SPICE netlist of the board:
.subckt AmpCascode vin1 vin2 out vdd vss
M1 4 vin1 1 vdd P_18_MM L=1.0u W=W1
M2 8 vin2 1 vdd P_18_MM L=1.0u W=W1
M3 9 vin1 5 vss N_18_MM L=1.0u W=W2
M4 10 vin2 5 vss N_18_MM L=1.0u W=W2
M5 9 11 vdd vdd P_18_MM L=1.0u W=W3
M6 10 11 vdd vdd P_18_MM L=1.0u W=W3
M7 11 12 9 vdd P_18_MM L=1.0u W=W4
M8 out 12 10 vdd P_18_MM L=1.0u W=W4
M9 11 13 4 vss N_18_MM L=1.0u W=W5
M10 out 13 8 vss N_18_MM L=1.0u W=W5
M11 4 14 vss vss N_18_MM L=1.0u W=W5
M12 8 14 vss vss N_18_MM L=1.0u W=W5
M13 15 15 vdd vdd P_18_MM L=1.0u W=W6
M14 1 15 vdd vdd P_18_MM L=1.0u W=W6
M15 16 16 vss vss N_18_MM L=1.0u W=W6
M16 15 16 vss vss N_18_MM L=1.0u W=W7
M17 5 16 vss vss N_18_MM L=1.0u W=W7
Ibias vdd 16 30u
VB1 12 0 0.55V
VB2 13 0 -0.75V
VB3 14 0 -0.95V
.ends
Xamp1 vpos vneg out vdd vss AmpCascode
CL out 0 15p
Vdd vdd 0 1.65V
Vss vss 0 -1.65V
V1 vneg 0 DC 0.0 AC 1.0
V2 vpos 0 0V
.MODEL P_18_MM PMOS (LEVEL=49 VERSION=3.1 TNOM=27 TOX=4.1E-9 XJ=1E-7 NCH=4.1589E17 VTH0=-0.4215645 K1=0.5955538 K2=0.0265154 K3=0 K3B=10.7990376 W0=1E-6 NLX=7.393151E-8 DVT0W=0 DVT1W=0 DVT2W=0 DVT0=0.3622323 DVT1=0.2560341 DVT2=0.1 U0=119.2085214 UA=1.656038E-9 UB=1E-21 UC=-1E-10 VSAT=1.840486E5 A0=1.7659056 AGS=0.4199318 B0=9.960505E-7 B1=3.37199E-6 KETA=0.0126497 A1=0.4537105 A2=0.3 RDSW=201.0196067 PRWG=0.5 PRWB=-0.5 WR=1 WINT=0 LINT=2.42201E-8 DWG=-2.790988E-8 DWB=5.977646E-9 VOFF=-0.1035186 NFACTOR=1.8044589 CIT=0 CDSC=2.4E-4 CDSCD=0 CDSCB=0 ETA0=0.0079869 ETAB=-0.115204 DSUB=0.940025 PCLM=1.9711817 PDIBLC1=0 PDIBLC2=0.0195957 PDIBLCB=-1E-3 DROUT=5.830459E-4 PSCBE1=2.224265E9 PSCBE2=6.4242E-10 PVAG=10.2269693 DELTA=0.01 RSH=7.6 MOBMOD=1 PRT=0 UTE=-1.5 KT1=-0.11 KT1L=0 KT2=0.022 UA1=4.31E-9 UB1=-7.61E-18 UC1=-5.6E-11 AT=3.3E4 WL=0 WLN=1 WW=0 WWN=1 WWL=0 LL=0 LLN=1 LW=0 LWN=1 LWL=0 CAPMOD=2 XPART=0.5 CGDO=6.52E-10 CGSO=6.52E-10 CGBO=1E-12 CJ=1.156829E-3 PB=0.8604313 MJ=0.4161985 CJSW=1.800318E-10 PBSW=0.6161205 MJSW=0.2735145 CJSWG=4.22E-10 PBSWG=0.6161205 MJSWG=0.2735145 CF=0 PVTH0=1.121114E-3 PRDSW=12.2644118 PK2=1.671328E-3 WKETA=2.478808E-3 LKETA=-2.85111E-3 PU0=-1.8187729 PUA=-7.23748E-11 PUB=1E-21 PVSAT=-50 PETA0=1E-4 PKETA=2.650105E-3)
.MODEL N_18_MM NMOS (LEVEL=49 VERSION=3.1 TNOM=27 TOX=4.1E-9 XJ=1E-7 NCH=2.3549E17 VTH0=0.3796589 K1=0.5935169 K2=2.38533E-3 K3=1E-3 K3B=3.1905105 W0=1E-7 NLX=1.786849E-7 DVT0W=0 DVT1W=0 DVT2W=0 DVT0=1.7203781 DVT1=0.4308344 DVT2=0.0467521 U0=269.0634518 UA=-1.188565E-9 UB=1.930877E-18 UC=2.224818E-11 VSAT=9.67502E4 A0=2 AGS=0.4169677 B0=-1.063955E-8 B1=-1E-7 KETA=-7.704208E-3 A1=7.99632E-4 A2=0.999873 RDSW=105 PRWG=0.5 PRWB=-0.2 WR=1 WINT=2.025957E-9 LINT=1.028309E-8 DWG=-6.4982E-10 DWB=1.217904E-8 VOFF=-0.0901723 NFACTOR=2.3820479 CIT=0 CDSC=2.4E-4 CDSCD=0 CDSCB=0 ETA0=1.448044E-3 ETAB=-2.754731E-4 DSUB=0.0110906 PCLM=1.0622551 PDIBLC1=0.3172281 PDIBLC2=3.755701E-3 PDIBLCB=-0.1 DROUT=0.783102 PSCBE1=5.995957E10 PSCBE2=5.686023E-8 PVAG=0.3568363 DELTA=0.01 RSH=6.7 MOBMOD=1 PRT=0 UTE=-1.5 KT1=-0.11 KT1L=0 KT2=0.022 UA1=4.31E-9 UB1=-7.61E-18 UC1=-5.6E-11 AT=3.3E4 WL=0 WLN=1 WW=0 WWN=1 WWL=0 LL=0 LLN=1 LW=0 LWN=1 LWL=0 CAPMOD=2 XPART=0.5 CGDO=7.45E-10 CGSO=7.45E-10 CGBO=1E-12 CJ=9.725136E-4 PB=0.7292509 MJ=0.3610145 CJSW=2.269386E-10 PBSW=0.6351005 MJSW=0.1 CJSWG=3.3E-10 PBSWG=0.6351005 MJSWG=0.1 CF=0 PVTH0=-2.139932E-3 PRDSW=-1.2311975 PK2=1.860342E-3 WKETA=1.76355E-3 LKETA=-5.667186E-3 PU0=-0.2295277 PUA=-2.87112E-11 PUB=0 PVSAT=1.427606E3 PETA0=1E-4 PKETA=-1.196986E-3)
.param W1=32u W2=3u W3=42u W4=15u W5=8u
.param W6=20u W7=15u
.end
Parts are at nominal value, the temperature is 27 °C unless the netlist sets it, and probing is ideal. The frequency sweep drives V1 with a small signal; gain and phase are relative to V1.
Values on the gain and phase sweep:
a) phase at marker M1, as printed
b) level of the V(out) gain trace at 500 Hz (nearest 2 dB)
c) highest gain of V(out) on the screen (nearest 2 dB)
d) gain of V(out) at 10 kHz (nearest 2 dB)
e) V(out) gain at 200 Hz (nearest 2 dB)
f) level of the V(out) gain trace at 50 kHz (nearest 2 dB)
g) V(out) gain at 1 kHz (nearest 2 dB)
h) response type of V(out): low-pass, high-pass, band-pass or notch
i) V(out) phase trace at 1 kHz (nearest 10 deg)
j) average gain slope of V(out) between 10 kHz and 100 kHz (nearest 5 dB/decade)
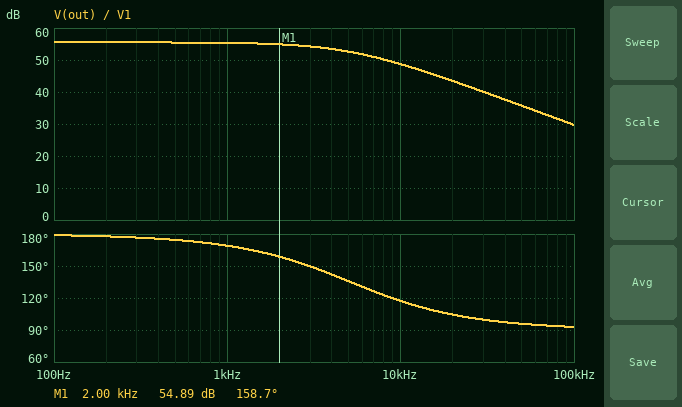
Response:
158.7 deg
56 dB
56 dB
48 dB
56 dB
36 dB
56 dB
low-pass
170 deg
-20 dB/decade
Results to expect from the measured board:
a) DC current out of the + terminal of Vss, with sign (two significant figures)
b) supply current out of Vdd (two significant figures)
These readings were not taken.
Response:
-200 µA
200 µA
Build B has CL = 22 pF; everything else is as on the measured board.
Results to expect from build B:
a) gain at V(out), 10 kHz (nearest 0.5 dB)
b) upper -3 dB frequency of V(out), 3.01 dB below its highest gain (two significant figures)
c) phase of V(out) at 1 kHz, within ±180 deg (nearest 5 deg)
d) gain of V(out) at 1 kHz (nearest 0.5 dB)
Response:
46.0 dB
3.5 kHz
165 deg
55.0 dB
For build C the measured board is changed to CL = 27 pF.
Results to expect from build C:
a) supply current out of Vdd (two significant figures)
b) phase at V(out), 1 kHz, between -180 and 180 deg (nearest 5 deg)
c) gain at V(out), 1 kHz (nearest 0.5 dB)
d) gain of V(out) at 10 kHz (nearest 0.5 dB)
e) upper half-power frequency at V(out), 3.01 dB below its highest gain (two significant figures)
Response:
200 µA
160 deg
55.0 dB
44.5 dB
2.9 kHz
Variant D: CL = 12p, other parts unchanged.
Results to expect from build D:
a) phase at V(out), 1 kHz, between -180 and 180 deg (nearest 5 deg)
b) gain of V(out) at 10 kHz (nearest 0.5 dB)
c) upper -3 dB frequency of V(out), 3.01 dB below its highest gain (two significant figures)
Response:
170 deg
50.0 dB
6.4 kHz
